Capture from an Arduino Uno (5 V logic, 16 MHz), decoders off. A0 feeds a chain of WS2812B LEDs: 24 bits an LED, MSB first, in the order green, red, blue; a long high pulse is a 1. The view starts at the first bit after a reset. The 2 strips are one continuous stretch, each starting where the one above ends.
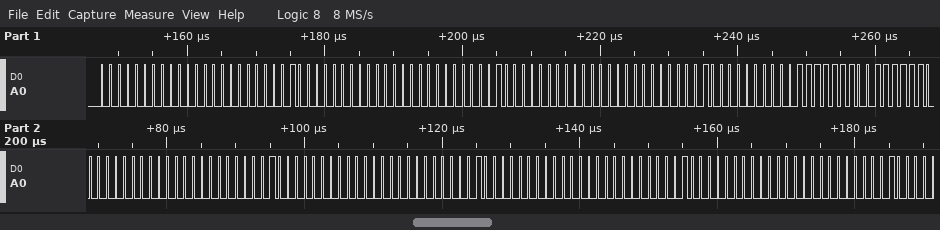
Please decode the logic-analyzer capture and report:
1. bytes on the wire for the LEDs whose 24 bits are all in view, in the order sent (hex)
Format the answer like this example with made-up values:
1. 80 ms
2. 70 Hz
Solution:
1. 00 00 02 00 00 02 00 00 02 00 7F 3F 00 00 02 00 00 02 00 00 02 00 00 02
